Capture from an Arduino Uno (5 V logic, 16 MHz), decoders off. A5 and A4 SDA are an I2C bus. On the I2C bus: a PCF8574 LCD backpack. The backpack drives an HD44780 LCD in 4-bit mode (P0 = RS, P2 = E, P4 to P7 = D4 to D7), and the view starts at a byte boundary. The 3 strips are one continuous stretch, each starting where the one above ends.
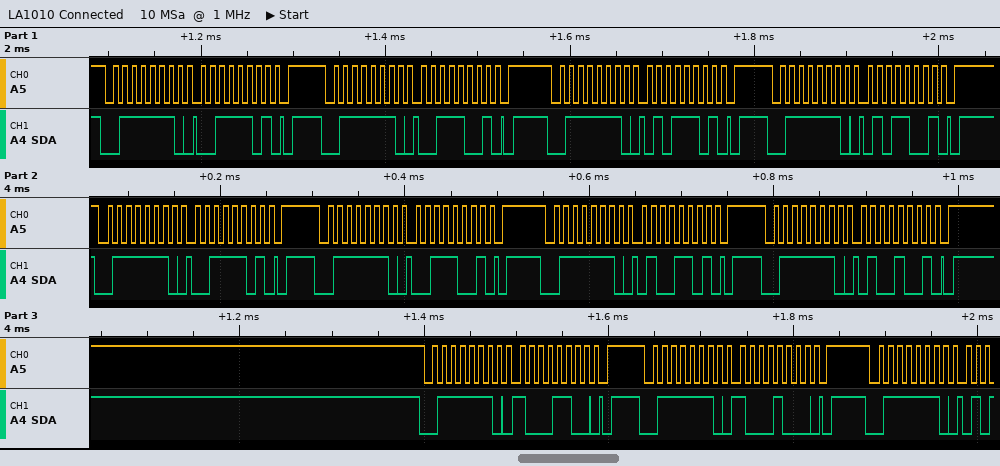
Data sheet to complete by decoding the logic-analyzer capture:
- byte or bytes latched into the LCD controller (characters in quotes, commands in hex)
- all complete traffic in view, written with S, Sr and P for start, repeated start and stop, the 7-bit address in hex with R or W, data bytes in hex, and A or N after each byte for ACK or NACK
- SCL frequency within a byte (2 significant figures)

'5' '4'
S 3FW A 3D A P S 3FW A 39 A P S 3FW A 5D A P S 3FW A 59 A P S 3FW A 3D A P S 3FW A 39 A P S 3FW A 4D A P S 3FW A 49 A P S 3FW A 8C A P S 3FW A 88 A P S 3FW A
100 kHz
